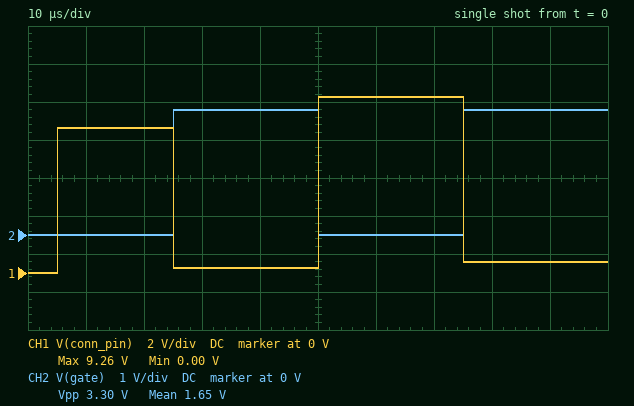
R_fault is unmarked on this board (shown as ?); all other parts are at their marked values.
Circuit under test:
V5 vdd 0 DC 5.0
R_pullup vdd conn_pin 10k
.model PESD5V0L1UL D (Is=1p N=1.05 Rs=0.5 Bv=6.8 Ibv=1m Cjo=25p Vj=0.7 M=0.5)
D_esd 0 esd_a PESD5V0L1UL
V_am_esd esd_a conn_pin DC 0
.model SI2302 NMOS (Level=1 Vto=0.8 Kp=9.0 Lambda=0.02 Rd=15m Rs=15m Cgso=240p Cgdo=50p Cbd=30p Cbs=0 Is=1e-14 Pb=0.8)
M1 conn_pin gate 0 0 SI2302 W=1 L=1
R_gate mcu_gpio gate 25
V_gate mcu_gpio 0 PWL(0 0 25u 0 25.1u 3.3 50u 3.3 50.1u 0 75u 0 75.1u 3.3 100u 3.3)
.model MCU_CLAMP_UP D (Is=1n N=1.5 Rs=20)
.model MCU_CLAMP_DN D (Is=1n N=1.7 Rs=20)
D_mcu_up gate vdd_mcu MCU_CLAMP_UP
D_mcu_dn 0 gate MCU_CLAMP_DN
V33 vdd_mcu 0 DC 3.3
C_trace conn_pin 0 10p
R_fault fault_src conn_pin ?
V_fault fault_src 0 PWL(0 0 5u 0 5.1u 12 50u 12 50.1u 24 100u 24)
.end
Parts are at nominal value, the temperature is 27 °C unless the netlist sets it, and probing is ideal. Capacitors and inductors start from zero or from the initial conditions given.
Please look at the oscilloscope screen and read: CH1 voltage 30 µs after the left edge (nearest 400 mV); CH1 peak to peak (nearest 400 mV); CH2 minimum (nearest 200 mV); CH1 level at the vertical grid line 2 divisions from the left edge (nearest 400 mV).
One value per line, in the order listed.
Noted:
400 mV
9.2 V
0 V
7.6 V
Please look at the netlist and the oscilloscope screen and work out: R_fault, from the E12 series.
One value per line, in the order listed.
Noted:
3.3 Ω
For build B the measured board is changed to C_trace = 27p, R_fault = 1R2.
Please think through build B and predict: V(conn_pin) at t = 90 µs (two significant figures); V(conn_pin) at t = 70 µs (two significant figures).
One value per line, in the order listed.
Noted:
1.8 V
12 V
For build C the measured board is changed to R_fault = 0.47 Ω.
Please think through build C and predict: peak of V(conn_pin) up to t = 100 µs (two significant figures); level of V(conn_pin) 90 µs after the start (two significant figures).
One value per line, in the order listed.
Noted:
16 V
9.9 V
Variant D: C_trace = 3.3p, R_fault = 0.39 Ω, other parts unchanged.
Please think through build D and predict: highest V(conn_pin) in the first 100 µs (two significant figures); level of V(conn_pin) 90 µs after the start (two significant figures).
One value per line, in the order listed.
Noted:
17 V
11 V
